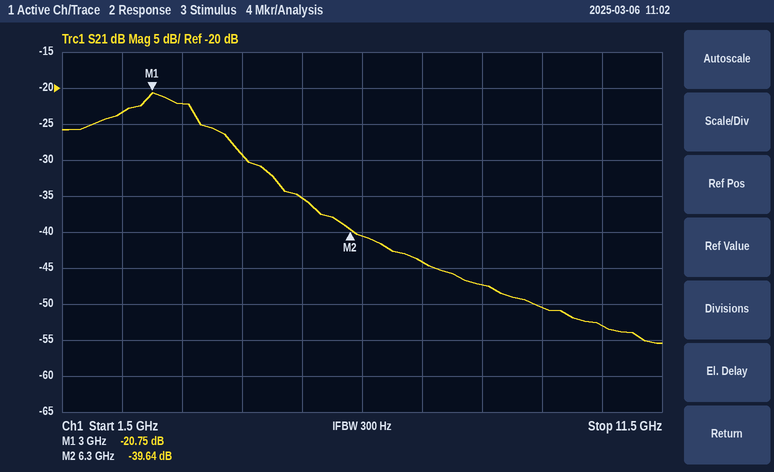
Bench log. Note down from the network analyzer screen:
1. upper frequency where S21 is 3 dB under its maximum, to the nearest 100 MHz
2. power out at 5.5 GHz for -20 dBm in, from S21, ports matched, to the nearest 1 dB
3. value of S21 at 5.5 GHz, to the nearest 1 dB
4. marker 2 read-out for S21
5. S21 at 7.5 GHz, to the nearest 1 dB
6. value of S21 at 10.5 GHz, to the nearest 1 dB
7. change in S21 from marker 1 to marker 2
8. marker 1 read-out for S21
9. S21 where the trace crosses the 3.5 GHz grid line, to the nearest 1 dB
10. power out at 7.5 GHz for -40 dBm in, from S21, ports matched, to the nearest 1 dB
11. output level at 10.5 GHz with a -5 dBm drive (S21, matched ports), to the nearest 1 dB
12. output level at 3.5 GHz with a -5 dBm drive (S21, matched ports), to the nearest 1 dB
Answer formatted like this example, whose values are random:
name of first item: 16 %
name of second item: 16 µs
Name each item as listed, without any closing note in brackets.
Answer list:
upper frequency where S21 is 3 dB under its maximum, to the nearest 100 MHz: 3.7 GHz
power out at 5.5 GHz for -20 dBm in, from S21, ports matched, to the nearest 1 dB: -55 dBm
value of S21 at 5.5 GHz, to the nearest 1 dB: -35 dB
marker 2 read-out for S21: -39.64 dB
S21 at 7.5 GHz, to the nearest 1 dB: -44 dB
value of S21 at 10.5 GHz, to the nearest 1 dB: -53 dB
change in S21 from marker 1 to marker 2: -18.89 dB
marker 1 read-out for S21: -20.75 dB
S21 where the trace crosses the 3.5 GHz grid line, to the nearest 1 dB: -22 dB
power out at 7.5 GHz for -40 dBm in, from S21, ports matched, to the nearest 1 dB: -84 dBm
output level at 10.5 GHz with a -5 dBm drive (S21, matched ports), to the nearest 1 dB: -58 dBm
output level at 3.5 GHz with a -5 dBm drive (S21, matched ports), to the nearest 1 dB: -27 dBm
